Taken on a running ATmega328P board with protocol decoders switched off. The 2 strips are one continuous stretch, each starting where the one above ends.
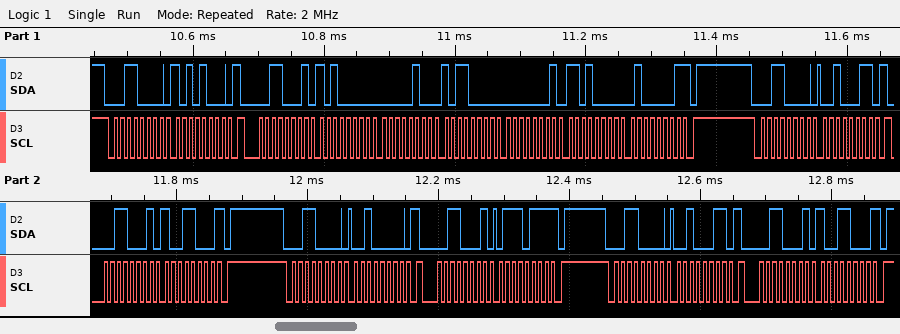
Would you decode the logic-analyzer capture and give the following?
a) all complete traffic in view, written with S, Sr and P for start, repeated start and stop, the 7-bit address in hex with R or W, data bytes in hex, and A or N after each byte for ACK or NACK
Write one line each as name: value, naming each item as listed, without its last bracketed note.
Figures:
all complete traffic in view, written with S, Sr and P for start, repeated start and stop, the 7-bit address in hex with R or W, data bytes in hex, and A or N after each byte for ACK or NACK: S 18W A A8 A Sr 18R A A0 A 04 A B0 A 01 A D0 A 41 N P S 18W A 23 A Sr 18R A 98 N P S 18W A 20 A Sr 18R A 77 N P S 18W A 23 A Sr 18R A 98 N P
